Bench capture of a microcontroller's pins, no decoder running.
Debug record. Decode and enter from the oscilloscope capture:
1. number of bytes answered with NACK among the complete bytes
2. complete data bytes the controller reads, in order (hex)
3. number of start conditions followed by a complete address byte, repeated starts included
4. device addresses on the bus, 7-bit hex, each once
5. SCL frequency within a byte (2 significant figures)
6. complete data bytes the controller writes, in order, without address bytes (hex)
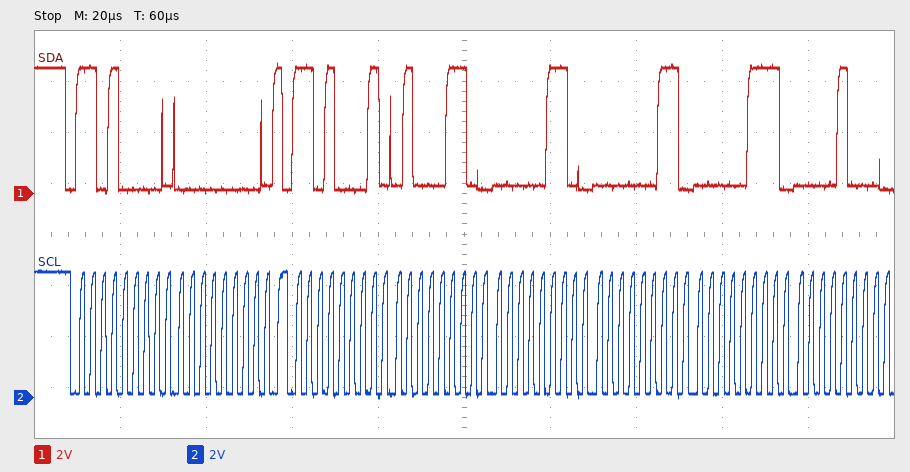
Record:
0
46 06 03 07 08
2
0x68
400 kHz
00
